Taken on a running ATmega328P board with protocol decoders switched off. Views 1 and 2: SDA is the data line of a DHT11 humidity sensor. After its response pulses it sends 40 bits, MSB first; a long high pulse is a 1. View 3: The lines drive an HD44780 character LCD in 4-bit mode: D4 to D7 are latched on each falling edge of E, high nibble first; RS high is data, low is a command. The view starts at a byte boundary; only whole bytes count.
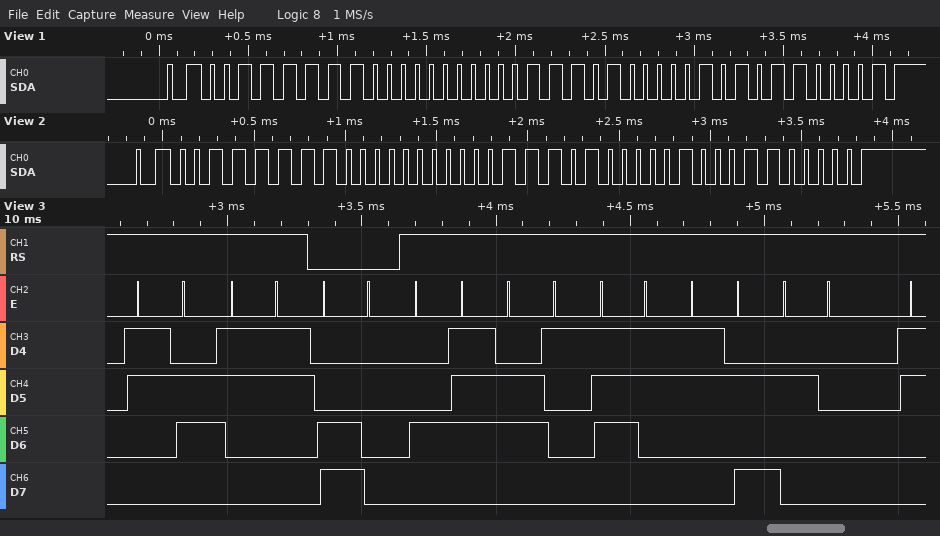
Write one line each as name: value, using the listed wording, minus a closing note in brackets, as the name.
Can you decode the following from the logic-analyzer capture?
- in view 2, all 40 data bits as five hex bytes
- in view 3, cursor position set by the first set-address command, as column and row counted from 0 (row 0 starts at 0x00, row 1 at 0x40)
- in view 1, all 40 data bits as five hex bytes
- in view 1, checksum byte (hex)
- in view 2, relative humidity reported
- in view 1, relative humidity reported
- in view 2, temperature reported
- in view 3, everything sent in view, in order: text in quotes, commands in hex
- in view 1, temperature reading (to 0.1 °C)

in view 2, all 40 data bits as five hex bytes: 3F 00 1D 04 60
in view 3, cursor position set by the first set-address command, as column and row counted from 0: column 0, row 1
in view 1, all 40 data bits as five hex bytes: 3F 00 1D 05 61
in view 1, checksum byte: 0x61
in view 2, relative humidity reported: 63 %
in view 1, relative humidity reported: 63 %
in view 2, temperature reported: 29.4 °C
in view 3, everything sent in view, in order: text in quotes, commands in hex: "63" 0xC0 "Gas: "
in view 1, temperature reading: 29.5 °C
